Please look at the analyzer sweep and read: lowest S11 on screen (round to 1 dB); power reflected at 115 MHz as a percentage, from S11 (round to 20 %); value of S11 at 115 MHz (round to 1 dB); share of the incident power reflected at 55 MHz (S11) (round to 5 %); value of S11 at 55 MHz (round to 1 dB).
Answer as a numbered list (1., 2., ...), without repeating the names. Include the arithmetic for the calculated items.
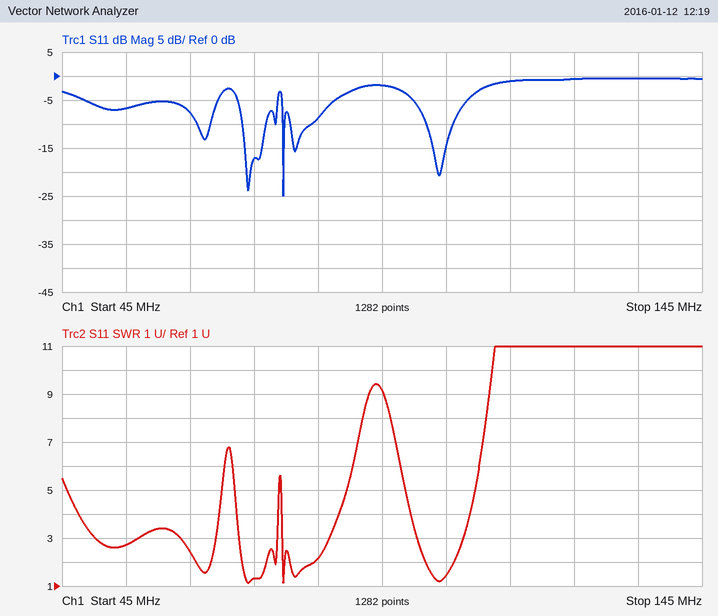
1. -25 dB
2. 10^(-1/10) ≈ 79.4 %, so 80 % to the nearest 20 %
3. -1 dB
4. 10^(-7/10) ≈ 20 %
5. -7 dB
